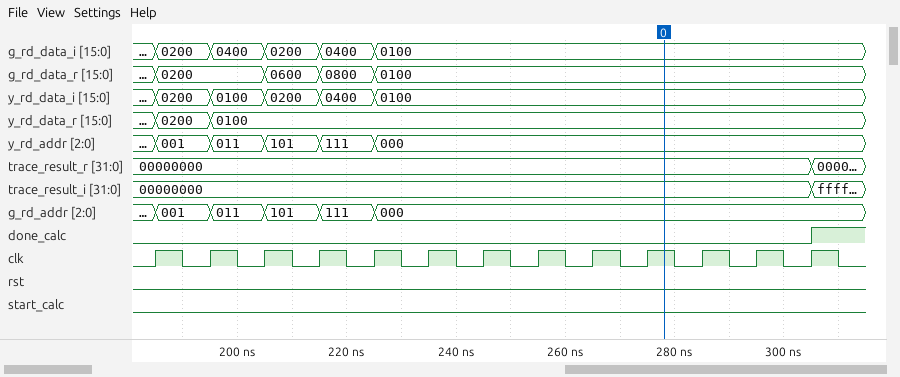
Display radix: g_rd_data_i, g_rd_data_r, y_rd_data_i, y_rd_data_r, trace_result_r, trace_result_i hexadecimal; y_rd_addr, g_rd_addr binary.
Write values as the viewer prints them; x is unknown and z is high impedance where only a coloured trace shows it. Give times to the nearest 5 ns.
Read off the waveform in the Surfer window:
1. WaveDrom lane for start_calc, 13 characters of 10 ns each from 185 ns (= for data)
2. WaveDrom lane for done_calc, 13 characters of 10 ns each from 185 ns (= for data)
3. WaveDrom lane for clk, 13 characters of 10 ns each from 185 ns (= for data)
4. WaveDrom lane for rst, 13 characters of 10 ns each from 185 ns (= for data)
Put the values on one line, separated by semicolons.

{name: 'start_calc', wave: '0............'}; {name: 'done_calc', wave: '0...........1'}; {name: 'clk', wave: 'p............'}; {name: 'rst', wave: '0............'}
